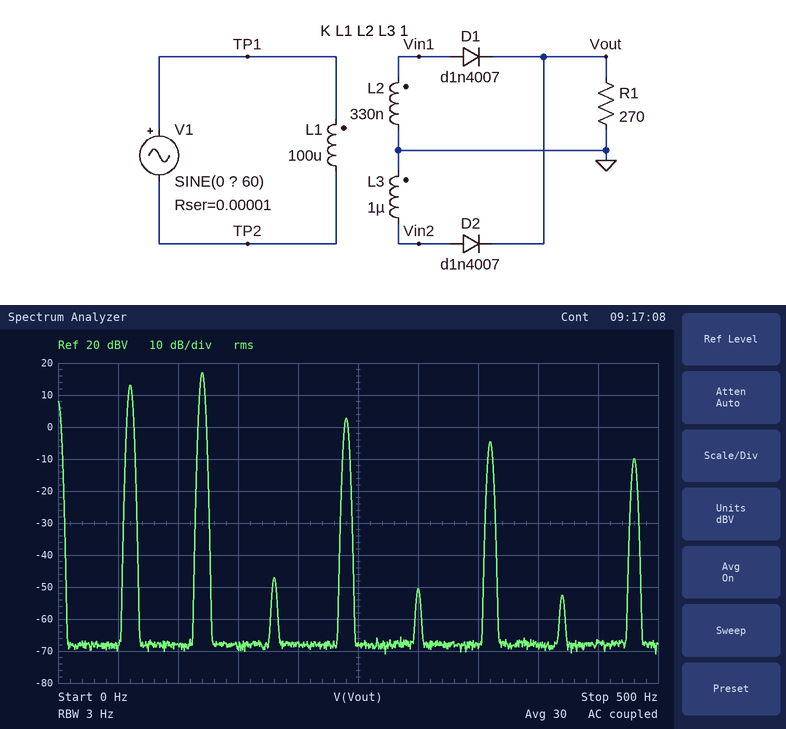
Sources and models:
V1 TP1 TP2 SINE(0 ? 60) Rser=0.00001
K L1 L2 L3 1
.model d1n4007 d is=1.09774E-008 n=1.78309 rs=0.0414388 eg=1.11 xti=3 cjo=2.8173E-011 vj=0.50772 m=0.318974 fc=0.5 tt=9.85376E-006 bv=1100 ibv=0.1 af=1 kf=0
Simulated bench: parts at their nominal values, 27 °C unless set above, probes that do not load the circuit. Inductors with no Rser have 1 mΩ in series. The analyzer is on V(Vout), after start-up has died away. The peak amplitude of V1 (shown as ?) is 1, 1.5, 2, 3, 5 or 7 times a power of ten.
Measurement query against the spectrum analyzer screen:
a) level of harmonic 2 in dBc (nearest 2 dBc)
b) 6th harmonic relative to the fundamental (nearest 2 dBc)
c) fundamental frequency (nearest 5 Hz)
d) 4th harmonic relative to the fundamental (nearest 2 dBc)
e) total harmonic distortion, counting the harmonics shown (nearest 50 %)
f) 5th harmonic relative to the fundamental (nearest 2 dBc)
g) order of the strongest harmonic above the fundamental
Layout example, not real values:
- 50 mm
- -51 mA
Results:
- 4 dBc
- -18 dBc
- 60 Hz
- -10 dBc
- 150 %
- -64 dBc
- 2
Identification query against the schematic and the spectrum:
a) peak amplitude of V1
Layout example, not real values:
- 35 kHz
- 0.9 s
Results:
- 300 V
